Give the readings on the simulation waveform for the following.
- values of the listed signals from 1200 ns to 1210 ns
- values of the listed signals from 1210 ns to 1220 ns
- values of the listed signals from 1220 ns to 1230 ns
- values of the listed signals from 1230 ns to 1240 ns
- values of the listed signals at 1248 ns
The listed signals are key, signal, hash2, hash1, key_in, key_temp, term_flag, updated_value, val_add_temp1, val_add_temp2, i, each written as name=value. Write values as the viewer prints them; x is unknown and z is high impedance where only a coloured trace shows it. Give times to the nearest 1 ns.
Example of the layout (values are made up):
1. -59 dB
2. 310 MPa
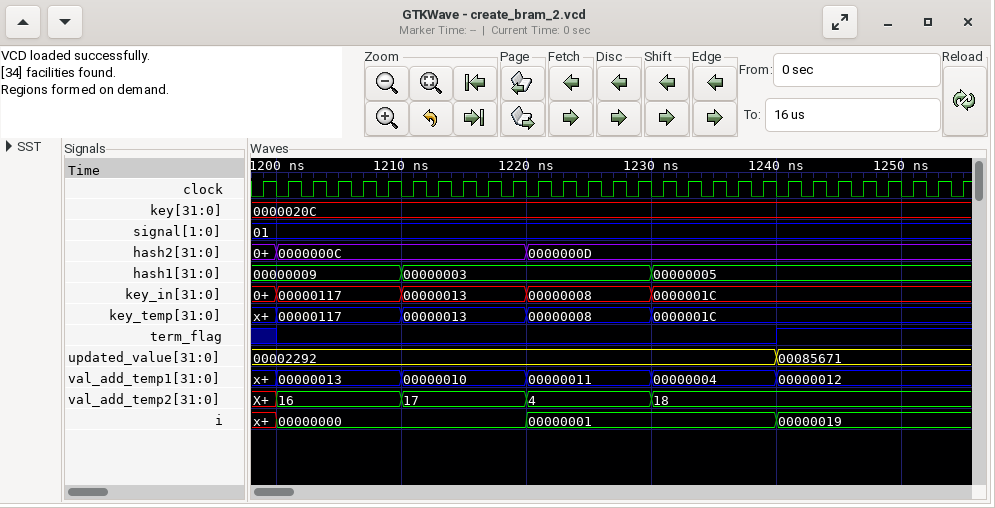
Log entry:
1. key=0000020C, signal=01, hash2=0000000C, hash1=00000009, key_in=00000117, key_temp=00000117, term_flag=0, updated_value=00002292, val_add_temp1=00000013, val_add_temp2=16, i=00000000
2. key=0000020C, signal=01, hash2=0000000C, hash1=00000003, key_in=00000013, key_temp=00000013, term_flag=0, updated_value=00002292, val_add_temp1=00000010, val_add_temp2=17, i=00000000
3. key=0000020C, signal=01, hash2=0000000D, hash1=00000003, key_in=00000008, key_temp=00000008, term_flag=0, updated_value=00002292, val_add_temp1=00000011, val_add_temp2=4, i=00000001
4. key=0000020C, signal=01, hash2=0000000D, hash1=00000005, key_in=0000001C, key_temp=0000001C, term_flag=0, updated_value=00002292, val_add_temp1=00000004, val_add_temp2=18, i=00000001
5. key=0000020C, signal=01, hash2=0000000D, hash1=00000005, key_in=0000001C, key_temp=0000001C, term_flag=1, updated_value=00085671, val_add_temp1=00000012, val_add_temp2=18, i=00000019
